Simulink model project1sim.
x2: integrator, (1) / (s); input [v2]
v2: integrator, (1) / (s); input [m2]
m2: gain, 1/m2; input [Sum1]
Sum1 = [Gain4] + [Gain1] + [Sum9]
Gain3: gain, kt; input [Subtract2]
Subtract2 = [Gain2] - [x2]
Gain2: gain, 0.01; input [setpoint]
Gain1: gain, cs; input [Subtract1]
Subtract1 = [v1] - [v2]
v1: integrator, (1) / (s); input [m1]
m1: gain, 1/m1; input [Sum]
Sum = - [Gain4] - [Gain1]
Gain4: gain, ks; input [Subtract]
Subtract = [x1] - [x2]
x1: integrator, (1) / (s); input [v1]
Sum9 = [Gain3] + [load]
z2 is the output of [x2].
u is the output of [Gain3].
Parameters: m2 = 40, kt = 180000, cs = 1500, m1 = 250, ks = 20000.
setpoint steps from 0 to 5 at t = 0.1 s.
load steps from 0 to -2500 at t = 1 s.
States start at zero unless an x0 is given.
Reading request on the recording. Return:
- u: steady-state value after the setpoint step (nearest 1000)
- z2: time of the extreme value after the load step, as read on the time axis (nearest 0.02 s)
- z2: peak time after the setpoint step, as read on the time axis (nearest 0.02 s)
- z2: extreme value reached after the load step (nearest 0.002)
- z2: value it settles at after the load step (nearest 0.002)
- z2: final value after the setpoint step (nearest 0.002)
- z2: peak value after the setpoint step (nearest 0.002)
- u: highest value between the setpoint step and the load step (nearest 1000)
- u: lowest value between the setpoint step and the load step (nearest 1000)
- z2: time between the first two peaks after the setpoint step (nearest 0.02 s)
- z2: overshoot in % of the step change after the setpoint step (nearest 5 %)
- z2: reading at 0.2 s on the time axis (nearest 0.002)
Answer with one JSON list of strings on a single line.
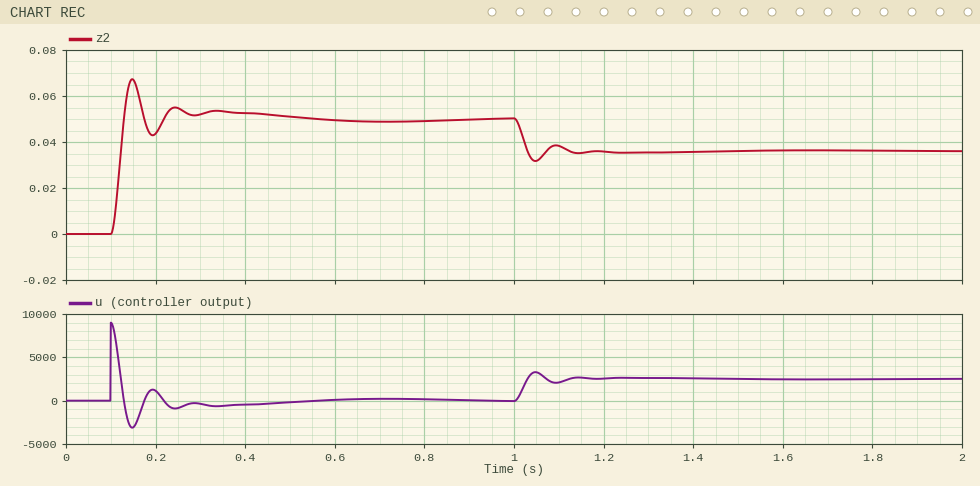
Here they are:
["0", "1.04 s", "0.14 s", "0.032", "0.036", "0.050", "0.068", "9000", "-3000", "0.10 s", "35 %", "0.044"]
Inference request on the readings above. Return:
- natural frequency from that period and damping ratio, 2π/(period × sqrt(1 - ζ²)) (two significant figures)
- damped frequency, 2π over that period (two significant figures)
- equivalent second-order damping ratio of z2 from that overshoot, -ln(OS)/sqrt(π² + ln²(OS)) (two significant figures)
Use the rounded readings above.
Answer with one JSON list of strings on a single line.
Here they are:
["66 rad/s", "63 rad/s", "0.32"]
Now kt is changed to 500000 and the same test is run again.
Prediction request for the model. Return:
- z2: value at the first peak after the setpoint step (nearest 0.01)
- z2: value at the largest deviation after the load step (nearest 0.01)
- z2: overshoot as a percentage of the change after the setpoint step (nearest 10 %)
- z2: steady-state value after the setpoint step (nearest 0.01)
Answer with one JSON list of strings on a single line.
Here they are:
["0.08", "0.04", "60 %", "0.05"]
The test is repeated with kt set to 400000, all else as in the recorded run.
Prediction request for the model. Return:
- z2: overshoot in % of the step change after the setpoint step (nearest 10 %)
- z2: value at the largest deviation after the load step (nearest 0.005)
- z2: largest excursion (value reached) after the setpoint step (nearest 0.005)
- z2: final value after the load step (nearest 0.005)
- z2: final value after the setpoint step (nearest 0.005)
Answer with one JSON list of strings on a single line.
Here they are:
["50 %", "0.040", "0.075", "0.045", "0.050"]
